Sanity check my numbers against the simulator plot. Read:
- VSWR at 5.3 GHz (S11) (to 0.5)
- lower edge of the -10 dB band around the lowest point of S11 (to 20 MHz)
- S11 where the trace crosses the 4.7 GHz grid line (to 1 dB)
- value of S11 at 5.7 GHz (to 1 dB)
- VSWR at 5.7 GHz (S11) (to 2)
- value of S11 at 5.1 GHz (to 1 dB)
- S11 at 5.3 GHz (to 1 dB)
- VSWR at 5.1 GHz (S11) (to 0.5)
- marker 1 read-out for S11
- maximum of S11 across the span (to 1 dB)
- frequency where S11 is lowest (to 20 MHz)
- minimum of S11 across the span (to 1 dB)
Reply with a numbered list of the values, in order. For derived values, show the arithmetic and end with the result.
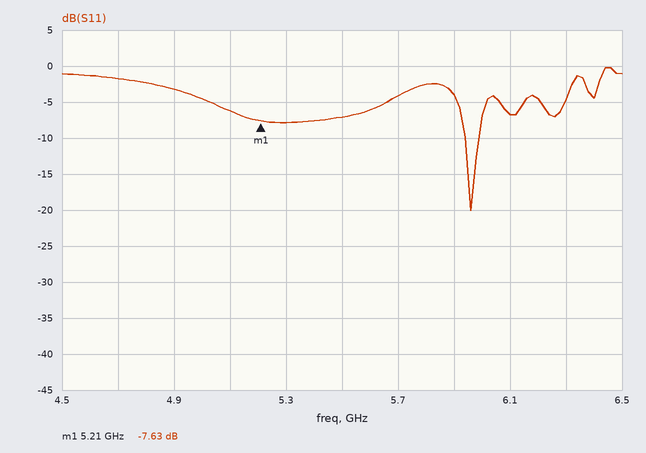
1. |Γ| = 10^(-8/20) = 0.3981; VSWR = (1 + 0.3981)/(1 − 0.3981) ≈ 2.32, so 2.5 to the nearest 0.5
2. 5.94 GHz
3. -2 dB
4. -4 dB
5. |Γ| = 10^(-4/20) = 0.6310; VSWR = (1 + 0.6310)/(1 − 0.6310) ≈ 4
6. -6 dB
7. -8 dB
8. |Γ| = 10^(-6/20) = 0.5012; VSWR = (1 + 0.5012)/(1 − 0.5012) ≈ 3.0
9. -7.63 dB
10. 0 dB
11. 5.96 GHz
12. -20 dB
